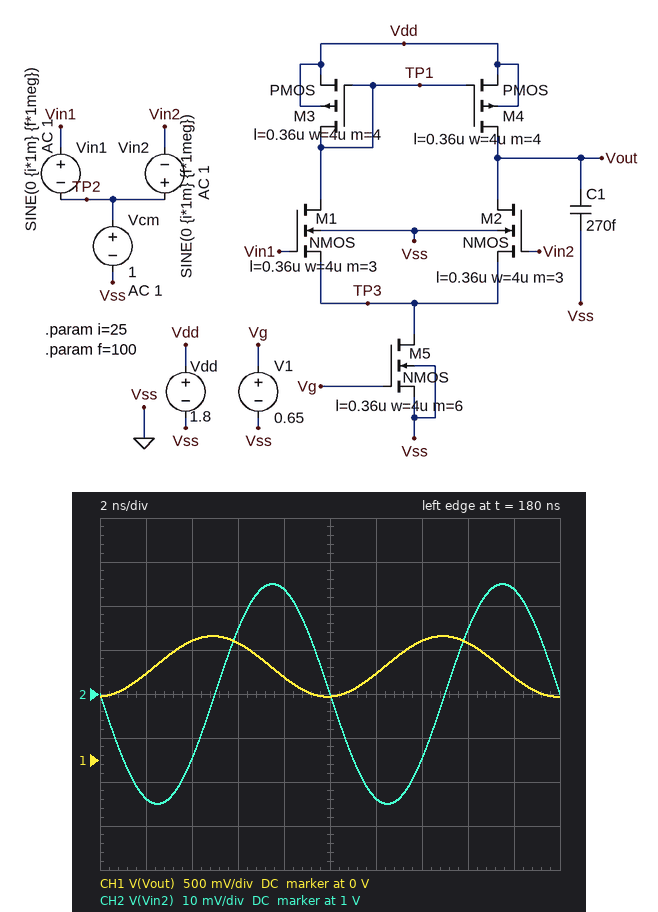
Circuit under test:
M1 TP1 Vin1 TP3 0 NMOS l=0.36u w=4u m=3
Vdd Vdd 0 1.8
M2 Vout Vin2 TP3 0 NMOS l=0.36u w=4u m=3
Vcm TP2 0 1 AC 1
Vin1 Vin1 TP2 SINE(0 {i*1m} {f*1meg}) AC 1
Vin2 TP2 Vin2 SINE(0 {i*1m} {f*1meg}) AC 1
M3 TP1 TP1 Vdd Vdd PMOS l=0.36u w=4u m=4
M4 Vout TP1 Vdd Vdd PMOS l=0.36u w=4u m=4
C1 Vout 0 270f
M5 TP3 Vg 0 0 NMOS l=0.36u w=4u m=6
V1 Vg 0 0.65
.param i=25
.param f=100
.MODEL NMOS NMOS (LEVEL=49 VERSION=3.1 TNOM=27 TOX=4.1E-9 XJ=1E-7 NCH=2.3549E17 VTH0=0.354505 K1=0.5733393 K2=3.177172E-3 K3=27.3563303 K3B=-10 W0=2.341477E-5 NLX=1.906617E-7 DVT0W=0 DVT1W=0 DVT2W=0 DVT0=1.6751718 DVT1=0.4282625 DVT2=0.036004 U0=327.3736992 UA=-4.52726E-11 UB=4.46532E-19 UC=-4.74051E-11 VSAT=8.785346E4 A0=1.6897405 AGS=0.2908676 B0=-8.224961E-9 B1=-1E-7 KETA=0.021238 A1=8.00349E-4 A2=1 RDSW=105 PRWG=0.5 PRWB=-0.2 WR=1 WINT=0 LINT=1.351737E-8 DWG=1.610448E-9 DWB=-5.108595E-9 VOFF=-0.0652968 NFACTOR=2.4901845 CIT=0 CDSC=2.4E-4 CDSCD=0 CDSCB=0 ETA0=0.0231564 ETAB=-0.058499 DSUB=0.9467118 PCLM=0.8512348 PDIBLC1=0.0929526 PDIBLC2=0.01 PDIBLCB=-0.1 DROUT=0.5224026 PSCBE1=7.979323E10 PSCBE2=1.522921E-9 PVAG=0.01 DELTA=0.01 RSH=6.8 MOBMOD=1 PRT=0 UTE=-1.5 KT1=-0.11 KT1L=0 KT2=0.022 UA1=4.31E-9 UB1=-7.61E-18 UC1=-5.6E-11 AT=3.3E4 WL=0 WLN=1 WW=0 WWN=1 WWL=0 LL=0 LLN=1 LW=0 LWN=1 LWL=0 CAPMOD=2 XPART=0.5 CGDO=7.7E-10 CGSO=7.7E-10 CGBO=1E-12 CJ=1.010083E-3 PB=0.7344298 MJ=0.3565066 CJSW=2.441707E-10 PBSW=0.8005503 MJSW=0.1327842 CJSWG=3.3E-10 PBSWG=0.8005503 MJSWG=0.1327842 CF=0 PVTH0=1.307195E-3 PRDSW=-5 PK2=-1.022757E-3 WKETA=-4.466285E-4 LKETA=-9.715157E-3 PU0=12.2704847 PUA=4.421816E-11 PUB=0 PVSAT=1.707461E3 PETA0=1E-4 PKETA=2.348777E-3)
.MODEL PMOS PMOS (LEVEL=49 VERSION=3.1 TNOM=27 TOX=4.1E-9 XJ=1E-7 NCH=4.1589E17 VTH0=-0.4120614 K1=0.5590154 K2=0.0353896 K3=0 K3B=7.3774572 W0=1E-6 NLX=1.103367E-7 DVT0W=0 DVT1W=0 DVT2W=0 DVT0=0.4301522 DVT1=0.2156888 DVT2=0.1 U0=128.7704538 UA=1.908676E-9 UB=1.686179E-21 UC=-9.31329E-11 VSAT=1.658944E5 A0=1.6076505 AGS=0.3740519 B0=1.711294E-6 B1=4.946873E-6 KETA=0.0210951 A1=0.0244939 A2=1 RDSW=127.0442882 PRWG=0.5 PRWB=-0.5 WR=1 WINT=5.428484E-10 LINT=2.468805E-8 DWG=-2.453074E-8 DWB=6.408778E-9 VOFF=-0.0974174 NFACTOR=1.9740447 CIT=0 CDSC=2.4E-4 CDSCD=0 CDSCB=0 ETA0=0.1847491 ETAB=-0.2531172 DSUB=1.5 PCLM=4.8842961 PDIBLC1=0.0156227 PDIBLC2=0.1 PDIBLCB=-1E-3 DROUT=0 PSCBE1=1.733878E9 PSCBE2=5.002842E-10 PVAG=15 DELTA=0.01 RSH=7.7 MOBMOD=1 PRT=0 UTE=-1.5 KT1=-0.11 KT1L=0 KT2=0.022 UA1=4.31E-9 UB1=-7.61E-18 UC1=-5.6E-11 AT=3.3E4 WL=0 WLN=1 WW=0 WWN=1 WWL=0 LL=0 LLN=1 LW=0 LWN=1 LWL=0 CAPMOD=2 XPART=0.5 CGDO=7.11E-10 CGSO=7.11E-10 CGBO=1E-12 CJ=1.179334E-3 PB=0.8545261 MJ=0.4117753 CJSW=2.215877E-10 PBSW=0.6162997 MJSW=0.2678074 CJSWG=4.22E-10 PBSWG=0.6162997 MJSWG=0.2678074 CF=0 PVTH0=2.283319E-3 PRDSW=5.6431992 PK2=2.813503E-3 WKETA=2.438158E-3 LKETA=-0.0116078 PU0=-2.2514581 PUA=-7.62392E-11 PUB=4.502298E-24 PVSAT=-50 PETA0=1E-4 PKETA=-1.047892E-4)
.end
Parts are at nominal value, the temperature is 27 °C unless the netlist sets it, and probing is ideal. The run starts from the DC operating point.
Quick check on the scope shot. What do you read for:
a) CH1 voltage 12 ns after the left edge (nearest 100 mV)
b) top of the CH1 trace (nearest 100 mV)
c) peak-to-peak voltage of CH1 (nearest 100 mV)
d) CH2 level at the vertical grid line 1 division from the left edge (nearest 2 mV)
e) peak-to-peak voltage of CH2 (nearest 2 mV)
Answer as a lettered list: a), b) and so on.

a) 1.0 V
b) 1.4 V
c) 700 mV
d) 976 mV
e) 50 mV
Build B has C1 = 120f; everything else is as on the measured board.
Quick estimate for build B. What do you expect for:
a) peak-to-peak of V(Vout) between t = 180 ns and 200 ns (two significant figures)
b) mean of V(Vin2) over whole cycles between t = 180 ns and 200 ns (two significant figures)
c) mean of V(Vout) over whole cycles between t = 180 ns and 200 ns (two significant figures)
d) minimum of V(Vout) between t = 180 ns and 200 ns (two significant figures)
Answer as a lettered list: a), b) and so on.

a) 1.2 V
b) 1.0 V
c) 1.0 V
d) 400 mV
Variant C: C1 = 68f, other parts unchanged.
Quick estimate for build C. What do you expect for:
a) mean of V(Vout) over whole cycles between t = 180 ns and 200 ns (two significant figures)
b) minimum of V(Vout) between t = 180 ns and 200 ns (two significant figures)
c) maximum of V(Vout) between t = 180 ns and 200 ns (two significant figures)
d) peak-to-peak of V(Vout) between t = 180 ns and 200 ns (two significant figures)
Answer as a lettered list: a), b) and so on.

a) 1.0 V
b) 350 mV
c) 1.7 V
d) 1.3 V
